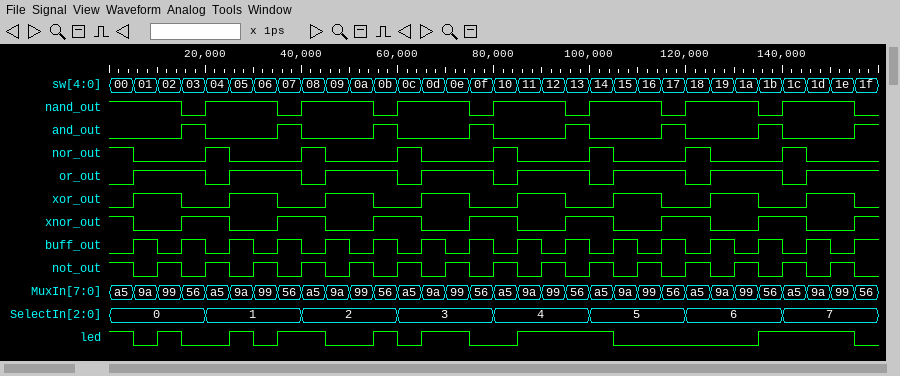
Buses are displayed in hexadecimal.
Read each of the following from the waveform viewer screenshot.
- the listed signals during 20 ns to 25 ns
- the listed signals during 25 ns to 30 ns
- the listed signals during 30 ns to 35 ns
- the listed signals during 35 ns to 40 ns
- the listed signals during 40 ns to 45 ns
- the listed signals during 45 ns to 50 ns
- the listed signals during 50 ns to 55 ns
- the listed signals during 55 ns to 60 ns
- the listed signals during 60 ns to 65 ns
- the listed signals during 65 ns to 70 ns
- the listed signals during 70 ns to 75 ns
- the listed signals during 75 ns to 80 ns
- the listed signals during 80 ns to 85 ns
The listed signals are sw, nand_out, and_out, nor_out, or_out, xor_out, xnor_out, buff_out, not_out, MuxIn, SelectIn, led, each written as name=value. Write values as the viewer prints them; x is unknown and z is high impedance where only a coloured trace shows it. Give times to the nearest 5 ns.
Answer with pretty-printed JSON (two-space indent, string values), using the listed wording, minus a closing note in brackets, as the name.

{
  "the listed signals during 20 ns to 25 ns": "sw=04, nand_out=1, and_out=0, nor_out=1, or_out=0, xor_out=0, xnor_out=1, buff_out=0, not_out=1, MuxIn=a5, SelectIn=1, led=0",
  "the listed signals during 25 ns to 30 ns": "sw=05, nand_out=1, and_out=0, nor_out=0, or_out=1, xor_out=1, xnor_out=0, buff_out=1, not_out=0, MuxIn=9a, SelectIn=1, led=1",
  "the listed signals during 30 ns to 35 ns": "sw=06, nand_out=1, and_out=0, nor_out=0, or_out=1, xor_out=1, xnor_out=0, buff_out=0, not_out=1, MuxIn=99, SelectIn=1, led=0",
  "the listed signals during 35 ns to 40 ns": "sw=07, nand_out=0, and_out=1, nor_out=0, or_out=1, xor_out=0, xnor_out=1, buff_out=1, not_out=0, MuxIn=56, SelectIn=1, led=1",
  "the listed signals during 40 ns to 45 ns": "sw=08, nand_out=1, and_out=0, nor_out=1, or_out=0, xor_out=0, xnor_out=1, buff_out=0, not_out=1, MuxIn=a5, SelectIn=2, led=1",
  "the listed signals during 45 ns to 50 ns": "sw=09, nand_out=1, and_out=0, nor_out=0, or_out=1, xor_out=1, xnor_out=0, buff_out=1, not_out=0, MuxIn=9a, SelectIn=2, led=0",
  "the listed signals during 50 ns to 55 ns": "sw=0a, nand_out=1, and_out=0, nor_out=0, or_out=1, xor_out=1, xnor_out=0, buff_out=0, not_out=1, MuxIn=99, SelectIn=2, led=0",
  "the listed signals during 55 ns to 60 ns": "sw=0b, nand_out=0, and_out=1, nor_out=0, or_out=1, xor_out=0, xnor_out=1, buff_out=1, not_out=0, MuxIn=56, SelectIn=2, led=1",
  "the listed signals during 60 ns to 65 ns": "sw=0c, nand_out=1, and_out=0, nor_out=1, or_out=0, xor_out=0, xnor_out=1, buff_out=0, not_out=1, MuxIn=a5, SelectIn=3, led=0",
  "the listed signals during 65 ns to 70 ns": "sw=0d, nand_out=1, and_out=0, nor_out=0, or_out=1, xor_out=1, xnor_out=0, buff_out=1, not_out=0, MuxIn=9a, SelectIn=3, led=1",
  "the listed signals during 70 ns to 75 ns": "sw=0e, nand_out=1, and_out=0, nor_out=0, or_out=1, xor_out=1, xnor_out=0, buff_out=0, not_out=1, MuxIn=99, SelectIn=3, led=1",
  "the listed signals during 75 ns to 80 ns": "sw=0f, nand_out=0, and_out=1, nor_out=0, or_out=1, xor_out=0, xnor_out=1, buff_out=1, not_out=0, MuxIn=56, SelectIn=3, led=0",
  "the listed signals during 80 ns to 85 ns": "sw=10, nand_out=1, and_out=0, nor_out=1, or_out=0, xor_out=0, xnor_out=1, buff_out=0, not_out=1, MuxIn=a5, SelectIn=4, led=0"
}
